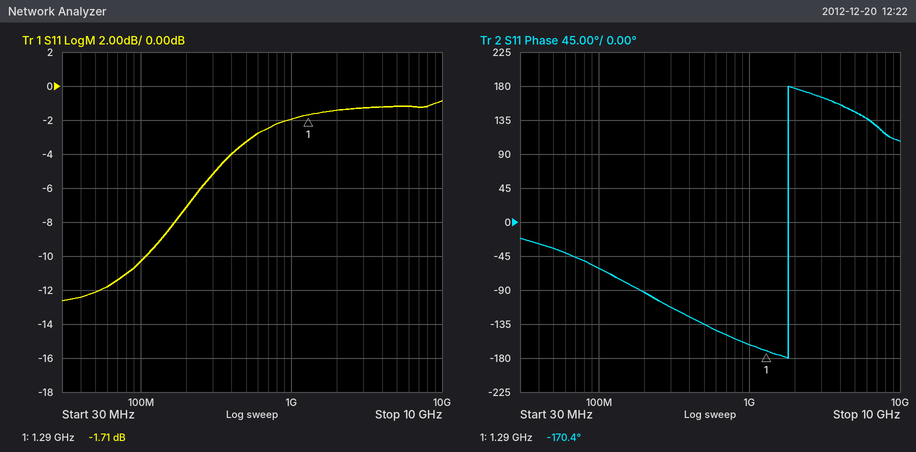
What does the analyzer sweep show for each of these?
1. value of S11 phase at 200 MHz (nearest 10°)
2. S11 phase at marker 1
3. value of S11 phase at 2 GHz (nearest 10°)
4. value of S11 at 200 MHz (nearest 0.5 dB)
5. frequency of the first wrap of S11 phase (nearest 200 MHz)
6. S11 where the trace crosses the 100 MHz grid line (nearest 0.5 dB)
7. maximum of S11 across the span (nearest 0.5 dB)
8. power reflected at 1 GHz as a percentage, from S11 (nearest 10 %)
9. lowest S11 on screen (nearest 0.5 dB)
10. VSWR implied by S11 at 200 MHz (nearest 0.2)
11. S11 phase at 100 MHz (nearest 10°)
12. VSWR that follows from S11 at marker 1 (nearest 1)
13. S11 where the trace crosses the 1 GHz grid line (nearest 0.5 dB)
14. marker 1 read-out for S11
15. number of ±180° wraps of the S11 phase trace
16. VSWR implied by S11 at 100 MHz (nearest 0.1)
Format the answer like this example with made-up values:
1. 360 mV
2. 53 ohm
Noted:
1. -90°
2. -170.4°
3. 180°
4. -7.0 dB
5. 1.8 GHz
6. -10.5 dB
7. -1.0 dB
8. 60 %
9. -12.5 dB
10. 2.6
11. -60°
12. 10
13. -2.0 dB
14. -1.71 dB
15. 1
16. 1.9
